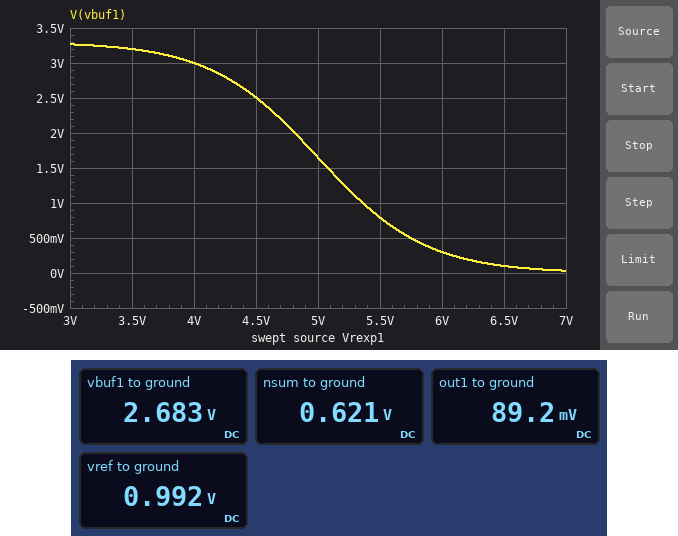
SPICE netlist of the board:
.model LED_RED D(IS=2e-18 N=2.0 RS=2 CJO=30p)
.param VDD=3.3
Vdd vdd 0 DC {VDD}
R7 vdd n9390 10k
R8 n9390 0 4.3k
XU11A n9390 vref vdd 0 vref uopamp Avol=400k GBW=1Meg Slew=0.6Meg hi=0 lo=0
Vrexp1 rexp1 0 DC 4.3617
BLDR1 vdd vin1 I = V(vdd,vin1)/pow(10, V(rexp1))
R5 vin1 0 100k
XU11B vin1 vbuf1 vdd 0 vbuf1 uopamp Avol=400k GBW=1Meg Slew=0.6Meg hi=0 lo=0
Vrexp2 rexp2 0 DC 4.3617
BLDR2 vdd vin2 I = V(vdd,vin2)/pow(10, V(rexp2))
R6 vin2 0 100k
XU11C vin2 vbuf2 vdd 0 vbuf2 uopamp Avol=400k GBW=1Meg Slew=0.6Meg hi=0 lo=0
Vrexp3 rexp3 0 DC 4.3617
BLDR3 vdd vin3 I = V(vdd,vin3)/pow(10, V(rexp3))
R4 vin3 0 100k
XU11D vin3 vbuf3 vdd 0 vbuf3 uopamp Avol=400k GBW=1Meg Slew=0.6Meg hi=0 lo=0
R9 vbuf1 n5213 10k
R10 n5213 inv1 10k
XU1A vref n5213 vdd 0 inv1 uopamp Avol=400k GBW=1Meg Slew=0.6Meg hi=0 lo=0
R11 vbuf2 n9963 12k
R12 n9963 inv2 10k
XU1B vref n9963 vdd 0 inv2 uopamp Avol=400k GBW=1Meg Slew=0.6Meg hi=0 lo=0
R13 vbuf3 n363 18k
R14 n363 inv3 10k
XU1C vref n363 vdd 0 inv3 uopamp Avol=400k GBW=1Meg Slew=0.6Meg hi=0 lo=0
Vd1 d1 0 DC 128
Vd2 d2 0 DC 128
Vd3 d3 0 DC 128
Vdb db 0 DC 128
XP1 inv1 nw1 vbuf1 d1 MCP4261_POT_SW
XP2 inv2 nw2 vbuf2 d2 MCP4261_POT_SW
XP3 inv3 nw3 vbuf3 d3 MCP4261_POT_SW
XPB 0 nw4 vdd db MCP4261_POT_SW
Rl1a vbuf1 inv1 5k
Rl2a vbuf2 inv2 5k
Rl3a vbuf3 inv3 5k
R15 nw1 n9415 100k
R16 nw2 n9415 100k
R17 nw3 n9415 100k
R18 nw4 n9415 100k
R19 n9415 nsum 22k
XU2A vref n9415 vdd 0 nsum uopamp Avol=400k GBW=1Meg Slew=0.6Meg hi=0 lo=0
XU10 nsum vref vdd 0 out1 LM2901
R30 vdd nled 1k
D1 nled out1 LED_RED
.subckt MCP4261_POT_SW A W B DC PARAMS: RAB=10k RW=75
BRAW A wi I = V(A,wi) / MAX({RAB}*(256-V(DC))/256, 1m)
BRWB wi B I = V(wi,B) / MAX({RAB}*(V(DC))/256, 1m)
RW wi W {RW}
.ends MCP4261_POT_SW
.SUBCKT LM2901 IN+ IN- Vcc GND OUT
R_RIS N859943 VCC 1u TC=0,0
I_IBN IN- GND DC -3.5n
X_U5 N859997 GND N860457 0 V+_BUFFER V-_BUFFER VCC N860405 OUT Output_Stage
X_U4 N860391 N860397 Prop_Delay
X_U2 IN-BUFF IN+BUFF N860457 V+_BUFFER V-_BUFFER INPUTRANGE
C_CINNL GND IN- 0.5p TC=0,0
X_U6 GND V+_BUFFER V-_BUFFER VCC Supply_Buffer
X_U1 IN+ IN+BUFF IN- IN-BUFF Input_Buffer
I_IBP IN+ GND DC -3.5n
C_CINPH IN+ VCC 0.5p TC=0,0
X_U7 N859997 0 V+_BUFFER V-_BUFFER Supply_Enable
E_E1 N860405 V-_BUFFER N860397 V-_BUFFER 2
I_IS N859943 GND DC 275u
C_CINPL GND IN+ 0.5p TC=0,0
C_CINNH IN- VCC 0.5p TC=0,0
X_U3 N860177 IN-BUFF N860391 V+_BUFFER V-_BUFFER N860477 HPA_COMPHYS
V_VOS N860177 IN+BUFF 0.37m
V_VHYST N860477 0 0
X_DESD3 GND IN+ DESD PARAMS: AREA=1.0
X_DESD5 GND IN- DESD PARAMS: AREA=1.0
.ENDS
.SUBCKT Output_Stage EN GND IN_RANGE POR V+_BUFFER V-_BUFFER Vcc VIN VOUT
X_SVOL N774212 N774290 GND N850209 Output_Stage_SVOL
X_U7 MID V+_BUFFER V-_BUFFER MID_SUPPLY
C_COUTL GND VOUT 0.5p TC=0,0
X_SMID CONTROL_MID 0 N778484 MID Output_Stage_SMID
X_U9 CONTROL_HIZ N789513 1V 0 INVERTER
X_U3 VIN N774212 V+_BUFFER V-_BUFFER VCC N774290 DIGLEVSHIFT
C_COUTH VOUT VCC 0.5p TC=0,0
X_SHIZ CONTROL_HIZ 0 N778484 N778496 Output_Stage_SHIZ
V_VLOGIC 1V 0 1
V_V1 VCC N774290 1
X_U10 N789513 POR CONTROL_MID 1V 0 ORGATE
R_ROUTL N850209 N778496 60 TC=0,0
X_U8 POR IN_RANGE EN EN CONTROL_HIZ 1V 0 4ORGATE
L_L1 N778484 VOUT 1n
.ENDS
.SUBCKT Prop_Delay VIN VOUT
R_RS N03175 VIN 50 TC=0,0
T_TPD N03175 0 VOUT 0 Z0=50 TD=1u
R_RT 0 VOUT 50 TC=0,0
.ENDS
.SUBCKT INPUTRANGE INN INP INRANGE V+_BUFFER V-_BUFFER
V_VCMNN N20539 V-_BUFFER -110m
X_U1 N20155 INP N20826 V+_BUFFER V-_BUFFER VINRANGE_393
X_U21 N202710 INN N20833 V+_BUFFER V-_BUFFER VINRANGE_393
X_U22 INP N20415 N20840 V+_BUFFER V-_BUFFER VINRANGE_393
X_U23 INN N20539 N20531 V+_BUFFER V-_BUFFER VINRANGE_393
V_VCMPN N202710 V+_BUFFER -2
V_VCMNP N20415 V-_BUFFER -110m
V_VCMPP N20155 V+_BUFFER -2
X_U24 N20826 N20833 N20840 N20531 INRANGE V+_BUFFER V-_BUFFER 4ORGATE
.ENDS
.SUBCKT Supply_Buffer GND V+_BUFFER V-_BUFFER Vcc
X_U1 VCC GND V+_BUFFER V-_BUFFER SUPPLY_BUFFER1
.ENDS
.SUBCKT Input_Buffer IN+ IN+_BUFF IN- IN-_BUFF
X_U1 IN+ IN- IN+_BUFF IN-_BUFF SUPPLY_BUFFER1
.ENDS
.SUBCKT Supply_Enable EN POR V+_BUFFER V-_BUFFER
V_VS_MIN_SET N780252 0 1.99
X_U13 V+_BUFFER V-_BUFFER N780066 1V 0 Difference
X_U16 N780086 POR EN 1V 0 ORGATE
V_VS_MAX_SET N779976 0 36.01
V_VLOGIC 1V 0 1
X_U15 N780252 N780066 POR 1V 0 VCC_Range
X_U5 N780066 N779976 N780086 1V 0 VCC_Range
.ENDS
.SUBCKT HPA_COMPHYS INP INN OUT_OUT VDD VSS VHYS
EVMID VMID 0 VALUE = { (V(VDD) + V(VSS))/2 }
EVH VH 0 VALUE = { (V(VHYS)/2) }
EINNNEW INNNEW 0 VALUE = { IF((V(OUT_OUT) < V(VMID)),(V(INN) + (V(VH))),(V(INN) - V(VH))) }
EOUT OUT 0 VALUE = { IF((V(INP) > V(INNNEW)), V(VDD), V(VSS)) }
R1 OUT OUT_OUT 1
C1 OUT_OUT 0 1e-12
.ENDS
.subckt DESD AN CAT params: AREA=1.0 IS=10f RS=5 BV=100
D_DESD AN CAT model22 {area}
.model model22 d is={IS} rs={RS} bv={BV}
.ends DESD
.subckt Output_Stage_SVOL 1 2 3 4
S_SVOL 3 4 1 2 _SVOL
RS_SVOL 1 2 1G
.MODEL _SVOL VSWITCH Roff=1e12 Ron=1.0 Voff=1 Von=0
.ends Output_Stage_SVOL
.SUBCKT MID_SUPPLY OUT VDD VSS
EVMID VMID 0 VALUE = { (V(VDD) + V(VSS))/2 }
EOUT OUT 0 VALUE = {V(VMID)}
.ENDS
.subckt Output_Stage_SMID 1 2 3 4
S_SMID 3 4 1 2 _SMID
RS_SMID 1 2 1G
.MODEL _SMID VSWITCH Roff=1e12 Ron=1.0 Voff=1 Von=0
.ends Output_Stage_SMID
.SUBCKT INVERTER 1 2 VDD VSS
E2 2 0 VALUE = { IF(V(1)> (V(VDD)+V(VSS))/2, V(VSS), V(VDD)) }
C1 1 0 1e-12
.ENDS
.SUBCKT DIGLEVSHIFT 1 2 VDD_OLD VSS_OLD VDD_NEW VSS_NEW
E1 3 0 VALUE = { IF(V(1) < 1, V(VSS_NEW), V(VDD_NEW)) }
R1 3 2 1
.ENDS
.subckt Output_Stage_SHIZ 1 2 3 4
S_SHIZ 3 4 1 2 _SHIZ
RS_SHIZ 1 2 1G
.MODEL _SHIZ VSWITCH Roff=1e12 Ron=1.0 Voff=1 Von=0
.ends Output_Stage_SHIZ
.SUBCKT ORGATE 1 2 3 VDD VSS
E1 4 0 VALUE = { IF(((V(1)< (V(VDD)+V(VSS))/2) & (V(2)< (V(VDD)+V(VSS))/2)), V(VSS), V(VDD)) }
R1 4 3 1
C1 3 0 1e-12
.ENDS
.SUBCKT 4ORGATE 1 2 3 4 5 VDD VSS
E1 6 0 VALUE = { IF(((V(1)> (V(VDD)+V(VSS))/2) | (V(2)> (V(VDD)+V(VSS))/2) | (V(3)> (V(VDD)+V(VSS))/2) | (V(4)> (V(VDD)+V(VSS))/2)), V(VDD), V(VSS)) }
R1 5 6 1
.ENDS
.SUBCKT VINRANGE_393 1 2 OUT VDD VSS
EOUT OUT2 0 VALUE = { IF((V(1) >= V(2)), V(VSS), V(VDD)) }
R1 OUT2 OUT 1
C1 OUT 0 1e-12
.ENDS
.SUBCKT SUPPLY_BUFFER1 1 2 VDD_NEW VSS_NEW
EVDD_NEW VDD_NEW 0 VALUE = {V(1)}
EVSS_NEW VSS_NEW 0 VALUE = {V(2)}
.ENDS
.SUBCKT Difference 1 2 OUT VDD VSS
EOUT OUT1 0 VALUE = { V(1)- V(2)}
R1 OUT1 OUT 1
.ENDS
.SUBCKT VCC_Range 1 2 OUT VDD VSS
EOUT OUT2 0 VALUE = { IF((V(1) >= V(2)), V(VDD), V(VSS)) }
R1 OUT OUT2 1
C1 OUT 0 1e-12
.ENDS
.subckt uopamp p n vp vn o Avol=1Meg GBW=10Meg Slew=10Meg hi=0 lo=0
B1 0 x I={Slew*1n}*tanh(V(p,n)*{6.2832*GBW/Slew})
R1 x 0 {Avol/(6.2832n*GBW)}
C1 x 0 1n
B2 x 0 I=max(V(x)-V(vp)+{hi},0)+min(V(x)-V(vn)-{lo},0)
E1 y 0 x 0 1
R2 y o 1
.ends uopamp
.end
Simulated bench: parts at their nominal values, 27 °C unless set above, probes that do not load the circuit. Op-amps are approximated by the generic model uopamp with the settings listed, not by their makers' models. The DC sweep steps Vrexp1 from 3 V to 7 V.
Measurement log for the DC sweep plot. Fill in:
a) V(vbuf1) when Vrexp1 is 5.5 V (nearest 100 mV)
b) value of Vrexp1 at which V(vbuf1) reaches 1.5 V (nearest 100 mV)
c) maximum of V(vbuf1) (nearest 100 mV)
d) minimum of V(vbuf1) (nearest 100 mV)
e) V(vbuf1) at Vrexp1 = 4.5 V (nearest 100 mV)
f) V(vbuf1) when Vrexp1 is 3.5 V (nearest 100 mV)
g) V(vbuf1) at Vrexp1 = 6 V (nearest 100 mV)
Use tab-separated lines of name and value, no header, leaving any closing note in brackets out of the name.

V(vbuf1) when Vrexp1 is 5.5 V	800 mV
value of Vrexp1 at which V(vbuf1) reaches 1.5 V	5.1 V
maximum of V(vbuf1)	3.3 V
minimum of V(vbuf1)	0 V
V(vbuf1) at Vrexp1 = 4.5 V	2.5 V
V(vbuf1) when Vrexp1 is 3.5 V	3.2 V
V(vbuf1) at Vrexp1 = 6 V	300 mV
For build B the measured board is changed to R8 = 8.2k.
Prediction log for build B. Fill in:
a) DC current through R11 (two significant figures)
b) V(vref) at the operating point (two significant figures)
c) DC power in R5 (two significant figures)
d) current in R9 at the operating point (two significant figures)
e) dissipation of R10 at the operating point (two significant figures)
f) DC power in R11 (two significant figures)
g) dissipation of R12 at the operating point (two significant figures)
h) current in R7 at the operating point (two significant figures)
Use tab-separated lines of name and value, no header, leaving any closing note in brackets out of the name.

DC current through R11	100 µA
V(vref) at the operating point	1.5 V
DC power in R5	72 µW
current in R9 at the operating point	120 µA
dissipation of R10 at the operating point	140 µW
DC power in R11	120 µW
dissipation of R12 at the operating point	99 µW
current in R7 at the operating point	180 µA
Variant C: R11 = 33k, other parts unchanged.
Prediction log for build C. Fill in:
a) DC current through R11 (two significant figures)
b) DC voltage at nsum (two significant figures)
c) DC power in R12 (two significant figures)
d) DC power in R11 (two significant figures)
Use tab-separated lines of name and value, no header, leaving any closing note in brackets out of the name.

DC current through R11	51 µA
DC voltage at nsum	570 mV
DC power in R12	26 µW
DC power in R11	87 µW
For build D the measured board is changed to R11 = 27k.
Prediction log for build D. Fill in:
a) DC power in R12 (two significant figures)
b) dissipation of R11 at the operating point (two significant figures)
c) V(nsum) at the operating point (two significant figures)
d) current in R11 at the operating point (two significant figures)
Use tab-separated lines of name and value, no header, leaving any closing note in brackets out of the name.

DC power in R12	39 µW
dissipation of R11 at the operating point	110 µW
V(nsum) at the operating point	580 mV
current in R11 at the operating point	63 µA
